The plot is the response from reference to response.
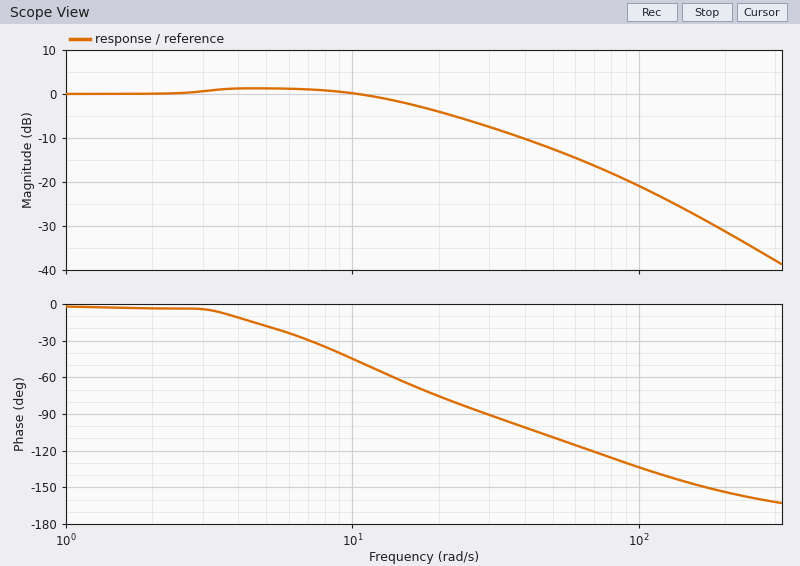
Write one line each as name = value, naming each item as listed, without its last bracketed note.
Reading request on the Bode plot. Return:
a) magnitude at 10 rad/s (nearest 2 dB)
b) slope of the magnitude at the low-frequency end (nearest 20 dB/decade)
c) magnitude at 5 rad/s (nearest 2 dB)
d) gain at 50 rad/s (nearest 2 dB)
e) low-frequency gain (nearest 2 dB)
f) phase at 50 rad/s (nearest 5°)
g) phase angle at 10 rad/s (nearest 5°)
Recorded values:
magnitude at 10 rad/s = 0 dB
slope of the magnitude at the low-frequency end = 0 dB/decade
magnitude at 5 rad/s = 2 dB
gain at 50 rad/s = -12 dB
low-frequency gain = 0 dB
phase at 50 rad/s = -110°
phase angle at 10 rad/s = -45°
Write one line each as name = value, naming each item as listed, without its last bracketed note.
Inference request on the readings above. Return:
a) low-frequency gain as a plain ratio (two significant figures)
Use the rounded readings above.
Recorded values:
low-frequency gain as a plain ratio = 1.0
